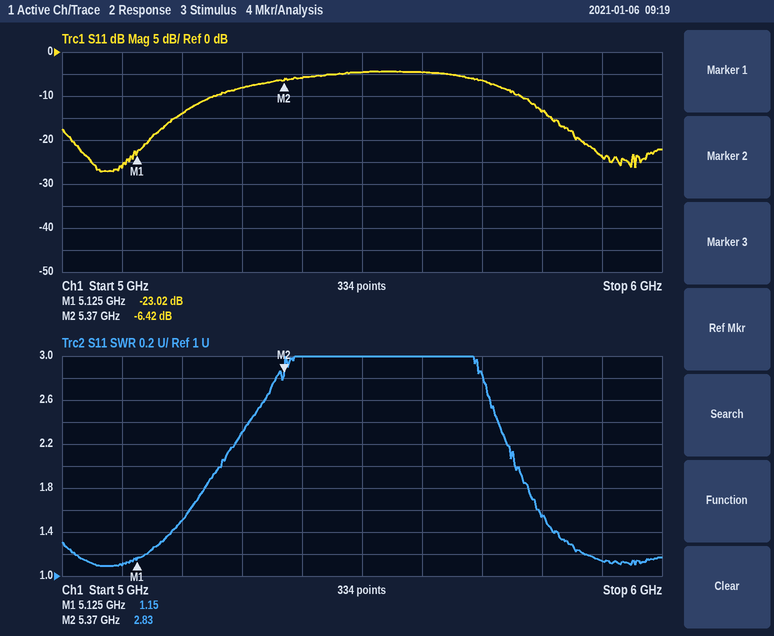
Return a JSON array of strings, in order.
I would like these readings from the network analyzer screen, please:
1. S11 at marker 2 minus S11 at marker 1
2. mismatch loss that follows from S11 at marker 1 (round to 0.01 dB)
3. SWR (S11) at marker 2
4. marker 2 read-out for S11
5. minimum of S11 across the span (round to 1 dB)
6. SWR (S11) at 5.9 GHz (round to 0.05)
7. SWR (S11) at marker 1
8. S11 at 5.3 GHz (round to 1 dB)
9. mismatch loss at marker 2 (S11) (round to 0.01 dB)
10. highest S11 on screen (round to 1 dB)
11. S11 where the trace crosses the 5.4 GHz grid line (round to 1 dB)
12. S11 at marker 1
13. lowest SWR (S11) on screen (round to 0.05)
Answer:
["16.60 dB", "0.02 dB", "2.83", "-6.42 dB", "-27 dB", "1.15", "1.15", "-8 dB", "1.12 dB", "-4 dB", "-6 dB", "-23.02 dB", "1.10"]
